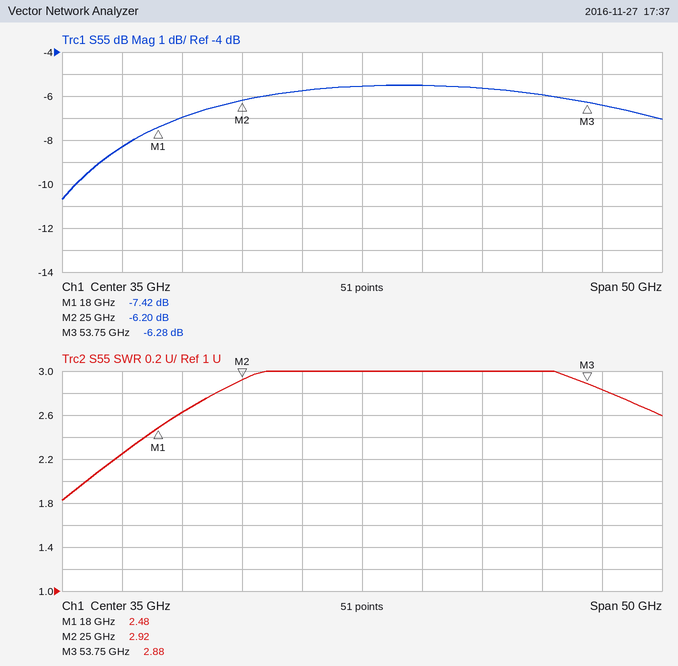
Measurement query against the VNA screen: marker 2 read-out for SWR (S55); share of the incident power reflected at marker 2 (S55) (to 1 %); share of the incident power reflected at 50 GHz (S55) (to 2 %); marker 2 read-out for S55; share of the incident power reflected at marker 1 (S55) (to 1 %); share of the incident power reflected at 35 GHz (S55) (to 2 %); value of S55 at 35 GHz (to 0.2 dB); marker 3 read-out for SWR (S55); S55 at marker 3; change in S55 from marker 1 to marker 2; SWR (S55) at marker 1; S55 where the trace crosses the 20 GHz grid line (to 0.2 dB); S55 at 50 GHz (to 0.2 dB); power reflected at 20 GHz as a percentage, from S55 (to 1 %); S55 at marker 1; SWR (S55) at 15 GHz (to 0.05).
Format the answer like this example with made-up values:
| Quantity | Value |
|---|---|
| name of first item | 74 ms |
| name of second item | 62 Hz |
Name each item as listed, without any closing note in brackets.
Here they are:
| Quantity | Value |
|---|---|
| marker 2 read-out for SWR | 2.92 |
| share of the incident power reflected at marker 2 (S55) | 24 % |
| share of the incident power reflected at 50 GHz (S55) | 26 % |
| marker 2 read-out for S55 | -6.20 dB |
| share of the incident power reflected at marker 1 (S55) | 18 % |
| share of the incident power reflected at 35 GHz (S55) | 28 % |
| value of S55 at 35 GHz | -5.6 dB |
| marker 3 read-out for SWR | 2.88 |
| S55 at marker 3 | -6.28 dB |
| change in S55 from marker 1 to marker 2 | 1.22 dB |
| SWR (S55) at marker 1 | 2.48 |
| S55 where the trace crosses the 20 GHz grid line | -7.0 dB |
| S55 at 50 GHz | -6.0 dB |
| power reflected at 20 GHz as a percentage, from S55 | 20 % |
| S55 at marker 1 | -7.42 dB |
| SWR (S55) at 15 GHz | 2.25 |
